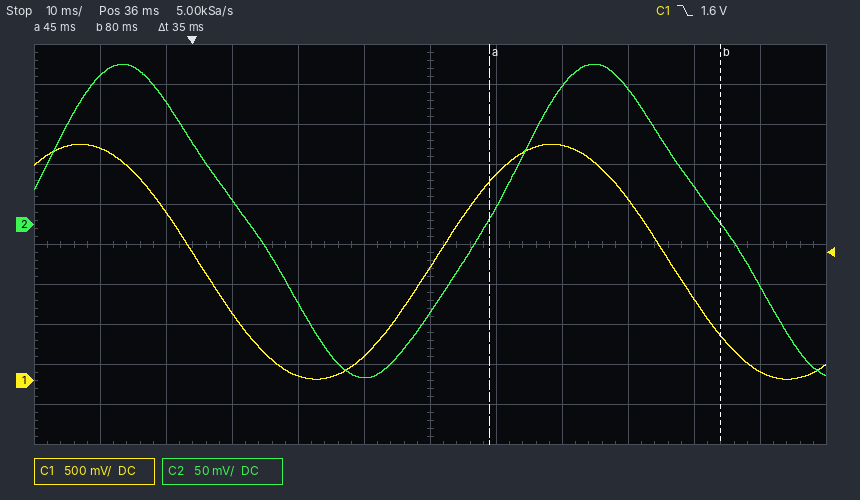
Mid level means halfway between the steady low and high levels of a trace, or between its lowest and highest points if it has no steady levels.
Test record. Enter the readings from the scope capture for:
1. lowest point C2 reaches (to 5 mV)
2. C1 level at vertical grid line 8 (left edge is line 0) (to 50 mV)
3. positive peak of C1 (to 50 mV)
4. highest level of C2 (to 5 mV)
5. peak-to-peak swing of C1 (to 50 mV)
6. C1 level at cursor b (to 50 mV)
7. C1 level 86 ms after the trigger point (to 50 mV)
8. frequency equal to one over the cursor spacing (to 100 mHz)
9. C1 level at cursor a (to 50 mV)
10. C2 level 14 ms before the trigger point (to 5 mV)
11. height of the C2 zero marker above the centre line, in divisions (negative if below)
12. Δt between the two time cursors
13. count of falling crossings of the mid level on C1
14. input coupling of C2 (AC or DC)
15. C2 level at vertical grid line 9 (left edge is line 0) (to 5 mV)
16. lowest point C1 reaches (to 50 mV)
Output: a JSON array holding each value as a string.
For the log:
["-190 mV", "2.95 V", "2.95 V", "200 mV", "2.95 V", "550 mV", "100 mV", "28.6 Hz", "2.50 V", "185 mV", "+0.5 div", "35 ms", "2", "DC", "170 mV", "0 mV"]
